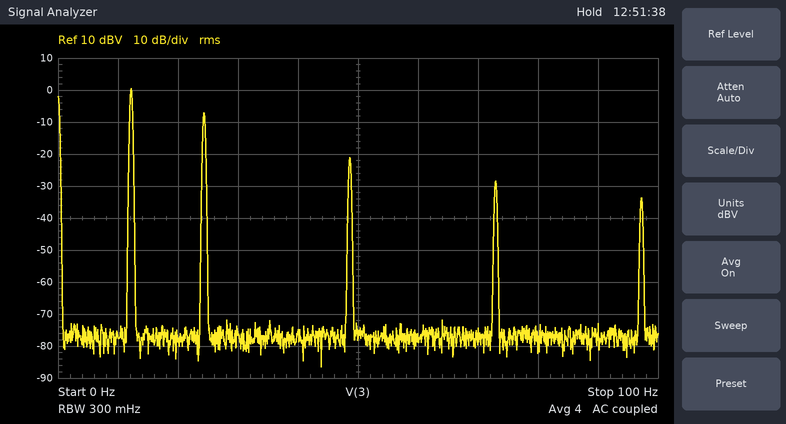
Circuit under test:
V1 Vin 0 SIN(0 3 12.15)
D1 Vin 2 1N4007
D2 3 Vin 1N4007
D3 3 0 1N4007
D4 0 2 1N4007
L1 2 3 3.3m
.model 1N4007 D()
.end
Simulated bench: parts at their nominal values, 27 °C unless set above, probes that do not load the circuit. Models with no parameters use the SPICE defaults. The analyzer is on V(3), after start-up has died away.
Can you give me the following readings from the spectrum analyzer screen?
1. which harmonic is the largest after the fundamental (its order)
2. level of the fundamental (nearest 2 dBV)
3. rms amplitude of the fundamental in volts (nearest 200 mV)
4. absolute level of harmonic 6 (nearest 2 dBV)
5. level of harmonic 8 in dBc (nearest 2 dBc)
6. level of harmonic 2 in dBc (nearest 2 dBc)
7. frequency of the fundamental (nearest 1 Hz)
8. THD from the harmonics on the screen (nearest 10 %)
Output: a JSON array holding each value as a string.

["2", "0 dBV", "1.0 V", "-28 dBV", "-34 dBc", "-8 dBc", "12 Hz", "40 %"]
